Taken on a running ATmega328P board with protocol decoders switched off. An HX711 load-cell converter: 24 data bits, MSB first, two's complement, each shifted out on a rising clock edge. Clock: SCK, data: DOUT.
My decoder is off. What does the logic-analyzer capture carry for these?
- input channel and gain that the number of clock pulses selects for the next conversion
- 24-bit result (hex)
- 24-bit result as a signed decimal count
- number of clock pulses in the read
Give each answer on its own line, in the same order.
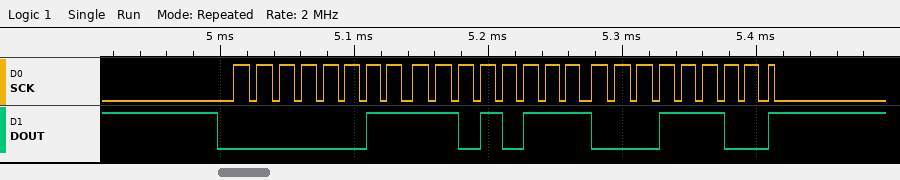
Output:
channel A, gain 128
0x03D71C
251676
25
